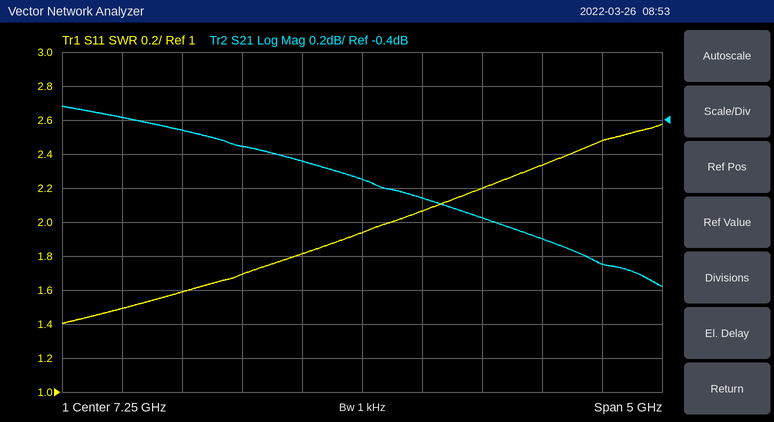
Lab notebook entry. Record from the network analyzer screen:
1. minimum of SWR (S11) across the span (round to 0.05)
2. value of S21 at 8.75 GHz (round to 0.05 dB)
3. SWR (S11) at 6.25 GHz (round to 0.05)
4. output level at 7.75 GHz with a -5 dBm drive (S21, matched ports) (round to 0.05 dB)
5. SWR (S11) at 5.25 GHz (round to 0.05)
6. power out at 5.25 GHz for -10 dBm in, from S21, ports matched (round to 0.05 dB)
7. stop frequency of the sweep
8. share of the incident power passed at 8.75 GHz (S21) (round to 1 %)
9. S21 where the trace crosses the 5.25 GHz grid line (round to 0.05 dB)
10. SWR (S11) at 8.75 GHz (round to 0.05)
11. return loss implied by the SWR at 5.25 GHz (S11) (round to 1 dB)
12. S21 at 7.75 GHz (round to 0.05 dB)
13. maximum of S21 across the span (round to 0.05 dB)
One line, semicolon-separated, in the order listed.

1.40; -1.10 dB; 1.70; -5.85 dBm; 1.50; -10.40 dBm; 9.75 GHz; 78 %; -0.40 dB; 2.35; 14 dB; -0.85 dB; -0.30 dB
